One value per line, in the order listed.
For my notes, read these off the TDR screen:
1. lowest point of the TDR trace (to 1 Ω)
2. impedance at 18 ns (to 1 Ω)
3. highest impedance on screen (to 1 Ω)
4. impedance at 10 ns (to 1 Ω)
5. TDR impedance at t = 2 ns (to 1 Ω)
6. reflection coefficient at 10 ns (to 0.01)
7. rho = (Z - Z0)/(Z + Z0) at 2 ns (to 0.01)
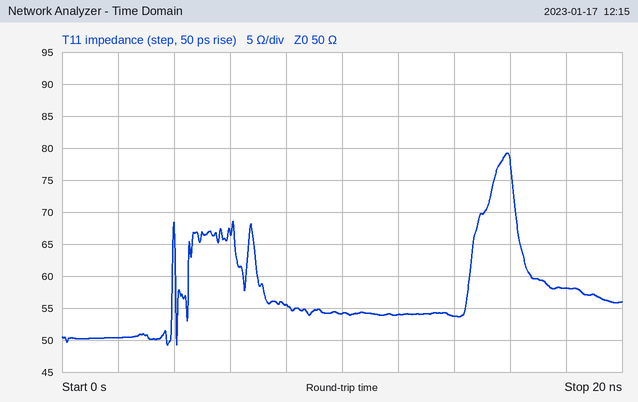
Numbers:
49 Ω
58 Ω
79 Ω
54 Ω
50 Ω
+0.04
0.00
